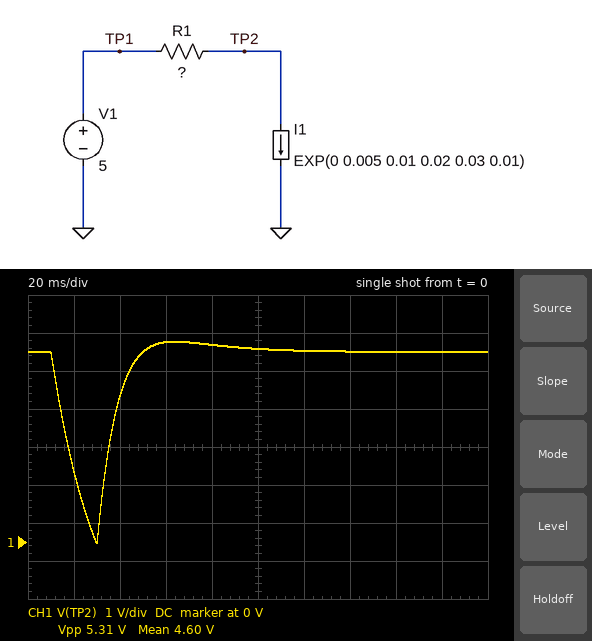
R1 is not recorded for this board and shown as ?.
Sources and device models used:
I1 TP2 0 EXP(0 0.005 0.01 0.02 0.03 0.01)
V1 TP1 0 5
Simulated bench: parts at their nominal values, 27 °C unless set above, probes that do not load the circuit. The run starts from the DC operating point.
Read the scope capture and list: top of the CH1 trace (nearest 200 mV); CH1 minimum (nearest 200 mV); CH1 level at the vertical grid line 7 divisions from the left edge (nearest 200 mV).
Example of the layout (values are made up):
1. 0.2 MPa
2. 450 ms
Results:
1. 5.2 V
2. 0 V
3. 5.0 V
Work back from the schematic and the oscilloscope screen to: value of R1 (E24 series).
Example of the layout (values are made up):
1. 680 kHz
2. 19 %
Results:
1. 1.6 kΩ
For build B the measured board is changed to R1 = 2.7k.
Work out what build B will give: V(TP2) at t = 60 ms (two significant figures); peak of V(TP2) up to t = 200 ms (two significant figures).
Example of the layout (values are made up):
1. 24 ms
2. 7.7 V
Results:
1. 5.4 V
2. 5.5 V
